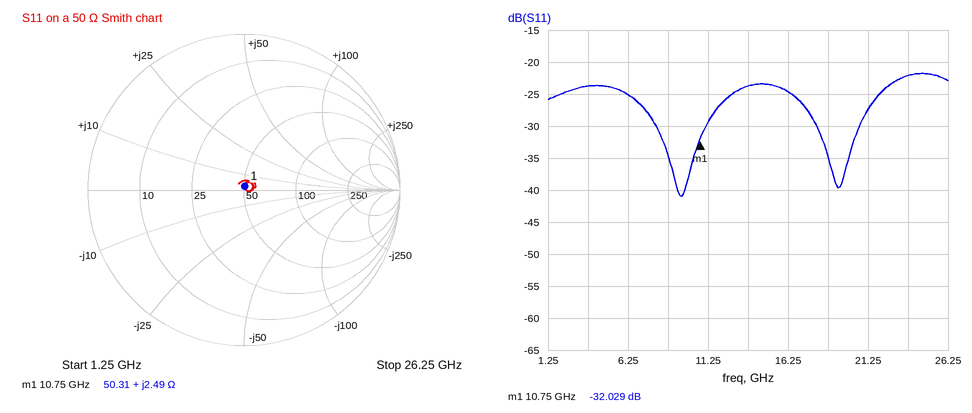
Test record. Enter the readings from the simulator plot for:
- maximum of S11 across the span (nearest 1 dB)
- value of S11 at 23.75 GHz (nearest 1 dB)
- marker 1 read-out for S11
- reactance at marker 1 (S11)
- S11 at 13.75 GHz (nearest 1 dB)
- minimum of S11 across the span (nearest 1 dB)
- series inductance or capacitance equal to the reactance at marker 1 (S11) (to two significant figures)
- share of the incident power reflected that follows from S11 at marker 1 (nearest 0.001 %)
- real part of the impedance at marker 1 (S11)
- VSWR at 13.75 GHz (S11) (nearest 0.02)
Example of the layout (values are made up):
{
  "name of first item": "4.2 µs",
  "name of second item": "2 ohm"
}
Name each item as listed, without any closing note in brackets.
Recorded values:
{
  "maximum of S11 across the span": "-22 dB",
  "value of S11 at 23.75 GHz": "-22 dB",
  "marker 1 read-out for S11": "-32.029 dB",
  "reactance at marker 1": "+2.49 Ω",
  "S11 at 13.75 GHz": "-24 dB",
  "minimum of S11 across the span": "-41 dB",
  "series inductance or capacitance equal to the reactance at marker 1 (S11)": "37 pH",
  "share of the incident power reflected that follows from S11 at marker 1": "0.063 %",
  "real part of the impedance at marker 1": "50.31 Ω",
  "VSWR at 13.75 GHz (S11)": "1.14"
}
